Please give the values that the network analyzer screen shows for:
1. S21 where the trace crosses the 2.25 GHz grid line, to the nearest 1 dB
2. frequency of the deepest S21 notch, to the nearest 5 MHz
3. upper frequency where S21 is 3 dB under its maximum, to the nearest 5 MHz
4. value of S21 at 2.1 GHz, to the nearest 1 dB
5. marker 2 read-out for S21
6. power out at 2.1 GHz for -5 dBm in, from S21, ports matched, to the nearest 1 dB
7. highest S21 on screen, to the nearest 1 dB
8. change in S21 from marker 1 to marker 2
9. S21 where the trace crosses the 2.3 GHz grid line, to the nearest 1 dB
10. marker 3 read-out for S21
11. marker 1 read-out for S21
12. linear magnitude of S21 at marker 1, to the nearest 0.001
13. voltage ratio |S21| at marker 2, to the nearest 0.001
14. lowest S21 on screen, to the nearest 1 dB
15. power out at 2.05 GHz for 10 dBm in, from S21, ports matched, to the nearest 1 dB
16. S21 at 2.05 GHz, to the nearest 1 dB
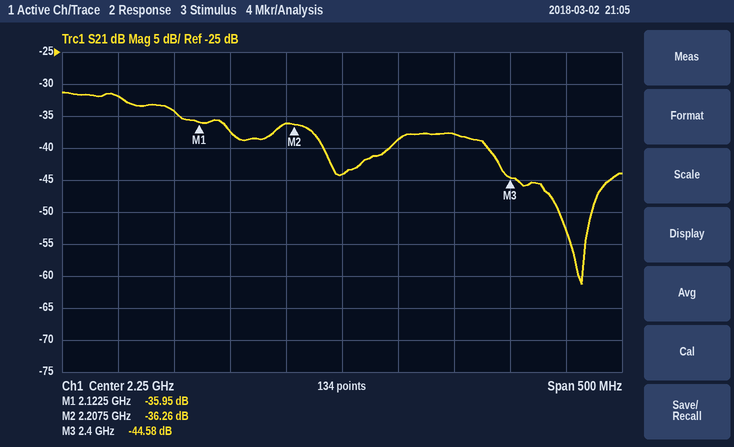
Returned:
-44 dB
2.465 GHz
2.100 GHz
-34 dB
-36.26 dB
-39 dBm
-31 dB
-0.31 dB
-39 dB
-44.58 dB
-35.95 dB
0.016
0.015
-61 dB
-22 dBm
-32 dB
